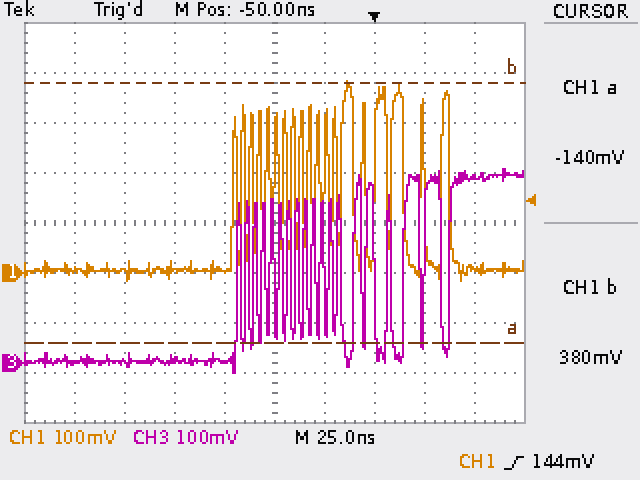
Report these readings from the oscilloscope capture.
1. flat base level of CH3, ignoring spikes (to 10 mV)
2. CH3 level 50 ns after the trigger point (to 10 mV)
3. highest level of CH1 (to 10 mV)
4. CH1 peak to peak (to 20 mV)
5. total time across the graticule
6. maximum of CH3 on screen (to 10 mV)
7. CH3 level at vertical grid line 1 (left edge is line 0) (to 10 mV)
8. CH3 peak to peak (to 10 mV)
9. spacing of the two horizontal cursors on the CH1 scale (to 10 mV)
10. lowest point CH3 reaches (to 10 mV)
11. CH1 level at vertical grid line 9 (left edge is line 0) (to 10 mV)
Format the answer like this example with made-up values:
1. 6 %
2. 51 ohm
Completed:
1. 0 mV
2. 370 mV
3. 380 mV
4. 400 mV
5. 250 ns
6. 390 mV
7. 0 mV
8. 410 mV
9. 520 mV
10. -20 mV
11. 10 mV
